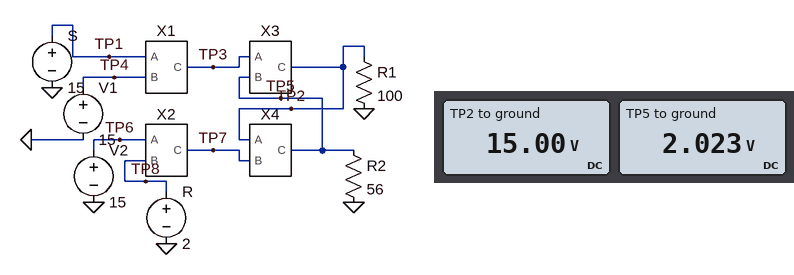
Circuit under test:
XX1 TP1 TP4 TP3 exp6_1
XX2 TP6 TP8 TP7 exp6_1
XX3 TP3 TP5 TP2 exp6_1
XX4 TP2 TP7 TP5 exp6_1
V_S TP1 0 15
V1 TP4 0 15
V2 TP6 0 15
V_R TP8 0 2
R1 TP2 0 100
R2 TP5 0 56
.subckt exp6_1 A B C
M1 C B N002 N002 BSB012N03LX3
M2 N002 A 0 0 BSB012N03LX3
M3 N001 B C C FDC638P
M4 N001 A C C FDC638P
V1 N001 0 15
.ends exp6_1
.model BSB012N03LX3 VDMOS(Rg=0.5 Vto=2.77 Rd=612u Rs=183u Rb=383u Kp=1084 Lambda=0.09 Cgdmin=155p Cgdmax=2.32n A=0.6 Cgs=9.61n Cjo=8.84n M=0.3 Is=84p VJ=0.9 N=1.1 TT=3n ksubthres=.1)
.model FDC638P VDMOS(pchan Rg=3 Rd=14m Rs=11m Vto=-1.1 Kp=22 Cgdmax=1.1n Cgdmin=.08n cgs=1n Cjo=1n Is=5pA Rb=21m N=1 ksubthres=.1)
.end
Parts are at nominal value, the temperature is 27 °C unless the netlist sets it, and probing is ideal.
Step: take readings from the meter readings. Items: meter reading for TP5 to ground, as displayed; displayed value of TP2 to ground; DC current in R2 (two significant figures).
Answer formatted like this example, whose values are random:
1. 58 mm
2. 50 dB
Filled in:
1. 2.023 V
2. 15.00 V
3. 36 mA
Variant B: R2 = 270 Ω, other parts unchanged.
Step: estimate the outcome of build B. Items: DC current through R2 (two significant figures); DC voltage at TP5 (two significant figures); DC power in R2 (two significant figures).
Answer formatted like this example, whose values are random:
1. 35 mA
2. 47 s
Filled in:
1. 7.5 mA
2. 2.0 V
3. 15 mW
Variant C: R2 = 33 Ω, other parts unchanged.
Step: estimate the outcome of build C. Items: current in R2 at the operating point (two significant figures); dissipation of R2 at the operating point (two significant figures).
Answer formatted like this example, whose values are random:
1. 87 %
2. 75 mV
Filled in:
1. 61 mA
2. 120 mW
